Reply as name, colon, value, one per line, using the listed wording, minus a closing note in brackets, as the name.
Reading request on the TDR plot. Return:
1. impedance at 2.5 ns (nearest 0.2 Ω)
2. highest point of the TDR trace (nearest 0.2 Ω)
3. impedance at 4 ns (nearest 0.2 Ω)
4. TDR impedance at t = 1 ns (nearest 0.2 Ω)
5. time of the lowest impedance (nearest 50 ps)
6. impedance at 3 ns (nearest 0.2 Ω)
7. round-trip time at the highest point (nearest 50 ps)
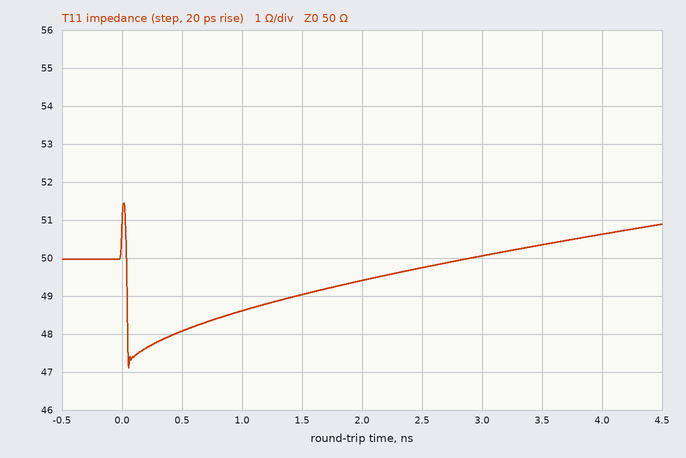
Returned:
impedance at 2.5 ns: 49.8 Ω
highest point of the TDR trace: 51.4 Ω
impedance at 4 ns: 50.6 Ω
TDR impedance at t = 1 ns: 48.6 Ω
time of the lowest impedance: 50 ps
impedance at 3 ns: 50.0 Ω
round-trip time at the highest point: 0 ps
